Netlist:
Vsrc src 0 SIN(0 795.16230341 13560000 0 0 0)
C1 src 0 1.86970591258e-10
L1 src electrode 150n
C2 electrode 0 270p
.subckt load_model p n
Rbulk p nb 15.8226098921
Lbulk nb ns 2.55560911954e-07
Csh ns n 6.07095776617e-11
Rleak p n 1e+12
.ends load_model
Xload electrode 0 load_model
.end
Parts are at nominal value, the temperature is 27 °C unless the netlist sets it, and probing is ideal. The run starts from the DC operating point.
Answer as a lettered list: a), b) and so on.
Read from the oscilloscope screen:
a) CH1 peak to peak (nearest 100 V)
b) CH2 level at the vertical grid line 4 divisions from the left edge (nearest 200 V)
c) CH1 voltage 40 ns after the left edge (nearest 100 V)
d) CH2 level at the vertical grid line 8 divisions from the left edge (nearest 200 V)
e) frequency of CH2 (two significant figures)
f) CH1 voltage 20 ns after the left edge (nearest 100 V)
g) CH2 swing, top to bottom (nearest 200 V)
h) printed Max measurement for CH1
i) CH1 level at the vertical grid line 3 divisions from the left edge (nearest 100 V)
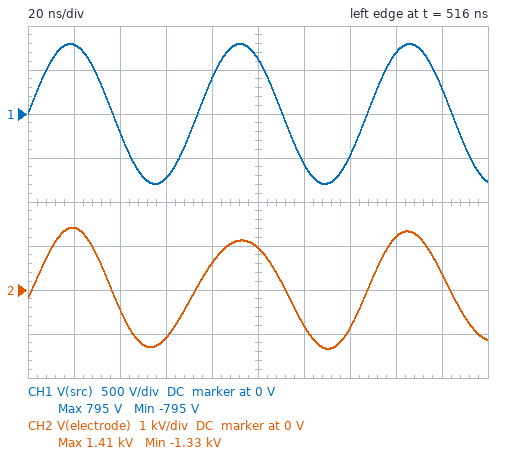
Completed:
a) 1.6 kV
b) 600 V
c) -200 V
d) 1.2 kV
e) 13 MHz
f) 800 V
g) 2.8 kV
h) 795 V
i) -700 V
